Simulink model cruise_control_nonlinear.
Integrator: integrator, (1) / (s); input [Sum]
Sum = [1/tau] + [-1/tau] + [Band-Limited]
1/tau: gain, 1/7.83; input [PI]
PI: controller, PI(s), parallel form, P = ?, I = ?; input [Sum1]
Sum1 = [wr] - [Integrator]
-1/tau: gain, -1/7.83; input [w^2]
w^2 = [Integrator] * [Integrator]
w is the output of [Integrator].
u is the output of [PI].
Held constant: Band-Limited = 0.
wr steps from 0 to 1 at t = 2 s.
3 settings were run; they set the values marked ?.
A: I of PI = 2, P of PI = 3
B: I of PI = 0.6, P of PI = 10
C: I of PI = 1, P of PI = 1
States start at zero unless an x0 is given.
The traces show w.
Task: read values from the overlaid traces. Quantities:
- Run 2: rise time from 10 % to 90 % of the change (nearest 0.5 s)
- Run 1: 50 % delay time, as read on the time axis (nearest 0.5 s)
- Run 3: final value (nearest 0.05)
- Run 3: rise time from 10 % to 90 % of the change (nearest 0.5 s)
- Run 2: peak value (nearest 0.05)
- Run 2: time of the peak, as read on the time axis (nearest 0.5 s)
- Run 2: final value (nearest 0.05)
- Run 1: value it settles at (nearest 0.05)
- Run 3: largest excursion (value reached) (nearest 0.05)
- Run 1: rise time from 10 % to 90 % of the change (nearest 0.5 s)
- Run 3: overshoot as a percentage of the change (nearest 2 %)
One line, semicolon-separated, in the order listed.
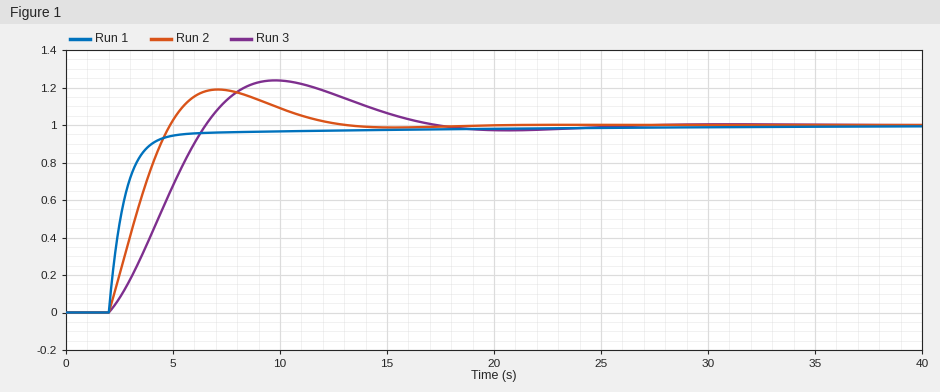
2.0 s; 2.5 s; 1.00; 3.5 s; 1.20; 7.0 s; 1.00; 1.00; 1.25; 2.0 s; 24 %
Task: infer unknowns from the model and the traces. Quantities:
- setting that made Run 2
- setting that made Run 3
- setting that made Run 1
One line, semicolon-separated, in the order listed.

A; C; B
